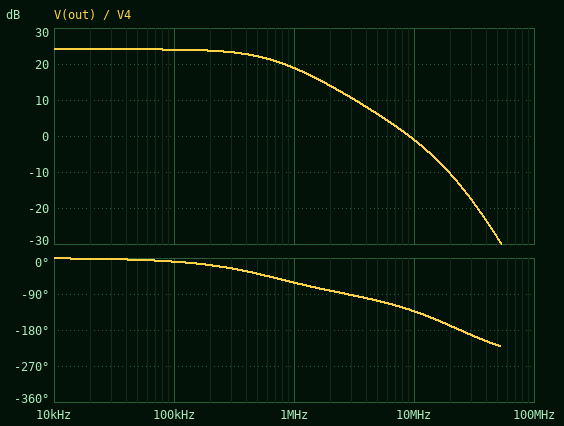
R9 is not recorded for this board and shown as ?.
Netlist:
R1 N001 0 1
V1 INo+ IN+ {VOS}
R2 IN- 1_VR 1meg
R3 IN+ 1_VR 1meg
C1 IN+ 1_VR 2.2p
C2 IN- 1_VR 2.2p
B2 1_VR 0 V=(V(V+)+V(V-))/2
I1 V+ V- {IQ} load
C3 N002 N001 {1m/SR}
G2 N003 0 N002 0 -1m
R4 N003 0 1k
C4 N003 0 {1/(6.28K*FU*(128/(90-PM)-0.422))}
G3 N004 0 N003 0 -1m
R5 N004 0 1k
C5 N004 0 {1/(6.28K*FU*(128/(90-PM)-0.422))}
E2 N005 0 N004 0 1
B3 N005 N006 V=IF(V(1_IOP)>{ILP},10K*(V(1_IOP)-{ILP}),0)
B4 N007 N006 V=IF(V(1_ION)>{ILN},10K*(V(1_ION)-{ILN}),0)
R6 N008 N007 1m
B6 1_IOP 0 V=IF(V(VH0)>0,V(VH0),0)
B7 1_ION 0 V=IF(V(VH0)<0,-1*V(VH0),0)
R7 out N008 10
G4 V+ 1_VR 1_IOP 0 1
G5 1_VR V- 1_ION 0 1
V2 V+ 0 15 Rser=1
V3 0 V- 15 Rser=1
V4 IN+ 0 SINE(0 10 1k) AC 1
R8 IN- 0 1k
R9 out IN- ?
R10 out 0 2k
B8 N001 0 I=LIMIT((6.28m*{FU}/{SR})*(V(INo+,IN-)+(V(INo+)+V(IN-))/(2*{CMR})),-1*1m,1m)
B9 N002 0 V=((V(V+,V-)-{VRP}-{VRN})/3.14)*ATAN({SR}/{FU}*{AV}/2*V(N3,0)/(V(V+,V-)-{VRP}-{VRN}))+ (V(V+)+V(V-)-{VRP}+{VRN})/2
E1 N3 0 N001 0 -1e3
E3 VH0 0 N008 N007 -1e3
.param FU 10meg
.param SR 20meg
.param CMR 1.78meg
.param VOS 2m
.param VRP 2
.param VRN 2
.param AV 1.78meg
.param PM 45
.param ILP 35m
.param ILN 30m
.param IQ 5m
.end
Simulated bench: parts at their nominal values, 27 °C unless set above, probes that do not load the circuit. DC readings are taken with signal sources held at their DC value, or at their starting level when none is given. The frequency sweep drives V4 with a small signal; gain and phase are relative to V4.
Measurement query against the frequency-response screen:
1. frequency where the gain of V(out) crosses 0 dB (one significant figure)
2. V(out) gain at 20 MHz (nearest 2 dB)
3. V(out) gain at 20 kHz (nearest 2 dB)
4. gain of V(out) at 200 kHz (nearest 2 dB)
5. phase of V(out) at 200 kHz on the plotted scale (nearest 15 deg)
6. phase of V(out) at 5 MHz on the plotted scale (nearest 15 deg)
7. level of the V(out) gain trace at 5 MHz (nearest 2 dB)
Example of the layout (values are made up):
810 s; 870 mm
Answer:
9 MHz; -10 dB; 24 dB; 24 dB; -15 deg; -105 deg; 6 dB
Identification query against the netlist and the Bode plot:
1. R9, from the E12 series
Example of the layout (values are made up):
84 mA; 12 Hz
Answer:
15 kΩ
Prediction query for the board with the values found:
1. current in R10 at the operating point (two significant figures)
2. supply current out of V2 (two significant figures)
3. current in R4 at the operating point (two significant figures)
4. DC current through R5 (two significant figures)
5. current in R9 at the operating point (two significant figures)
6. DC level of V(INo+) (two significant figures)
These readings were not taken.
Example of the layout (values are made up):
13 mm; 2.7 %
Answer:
16 µA; 5.0 mA; 32 µA; 32 µA; 2.0 µA; 2.0 mV
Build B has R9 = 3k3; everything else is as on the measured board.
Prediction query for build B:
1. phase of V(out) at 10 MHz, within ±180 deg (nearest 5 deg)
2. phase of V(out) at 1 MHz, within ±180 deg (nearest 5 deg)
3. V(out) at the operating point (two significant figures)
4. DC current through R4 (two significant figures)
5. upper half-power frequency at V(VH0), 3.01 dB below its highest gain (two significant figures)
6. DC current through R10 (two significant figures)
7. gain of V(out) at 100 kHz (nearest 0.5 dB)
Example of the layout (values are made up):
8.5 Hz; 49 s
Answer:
-125 deg; -25 deg; 8.6 mV; 8.7 µA; 3.0 MHz; 4.3 µA; 12.5 dB
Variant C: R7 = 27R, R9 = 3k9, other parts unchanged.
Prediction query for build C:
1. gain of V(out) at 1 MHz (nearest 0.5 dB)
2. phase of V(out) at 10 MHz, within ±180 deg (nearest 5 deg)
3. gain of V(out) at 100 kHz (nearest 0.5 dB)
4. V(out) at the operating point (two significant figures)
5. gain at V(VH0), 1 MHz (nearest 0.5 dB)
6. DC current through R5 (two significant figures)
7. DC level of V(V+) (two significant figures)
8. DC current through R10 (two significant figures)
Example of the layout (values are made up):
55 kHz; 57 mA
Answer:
13.0 dB; -130 deg; 14.0 dB; 9.8 mV; -50.0 dB; 10 µA; 15 V; 4.9 µA
